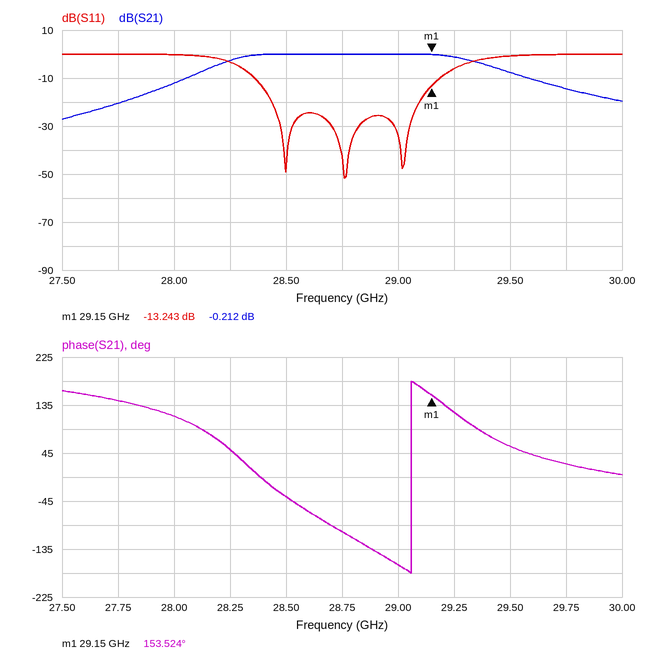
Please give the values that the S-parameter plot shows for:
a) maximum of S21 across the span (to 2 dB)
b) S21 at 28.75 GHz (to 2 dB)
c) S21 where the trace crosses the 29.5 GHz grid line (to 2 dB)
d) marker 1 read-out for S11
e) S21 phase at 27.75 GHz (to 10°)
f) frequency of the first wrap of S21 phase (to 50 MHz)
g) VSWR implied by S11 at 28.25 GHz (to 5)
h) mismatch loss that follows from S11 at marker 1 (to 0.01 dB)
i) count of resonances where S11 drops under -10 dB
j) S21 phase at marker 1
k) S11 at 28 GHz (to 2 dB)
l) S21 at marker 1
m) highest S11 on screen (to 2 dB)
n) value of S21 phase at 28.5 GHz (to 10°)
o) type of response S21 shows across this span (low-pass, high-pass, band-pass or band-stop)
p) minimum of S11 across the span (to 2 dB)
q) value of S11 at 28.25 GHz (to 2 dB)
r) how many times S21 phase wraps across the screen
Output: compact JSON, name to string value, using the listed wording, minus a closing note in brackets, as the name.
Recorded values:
{"maximum of S21 across the span": "0 dB", "S21 at 28.75 GHz": "0 dB", "S21 where the trace crosses the 29.5 GHz grid line": "-8 dB", "marker 1 read-out for S11": "-13.243 dB", "S21 phase at 27.75 GHz": "140°", "frequency of the first wrap of S21 phase": "29.05 GHz", "VSWR implied by S11 at 28.25 GHz": "5", "mismatch loss that follows from S11 at marker 1": "0.21 dB", "count of resonances where S11 drops under -10 dB": "3", "S21 phase at marker 1": "153.524°", "S11 at 28 GHz": "0 dB", "S21 at marker 1": "-0.212 dB", "highest S11 on screen": "0 dB", "value of S21 phase at 28.5 GHz": "-40°", "type of response S21 shows across this span": "band-pass", "minimum of S11 across the span": "-52 dB", "value of S11 at 28.25 GHz": "-4 dB", "how many times S21 phase wraps across the screen": "1"}
